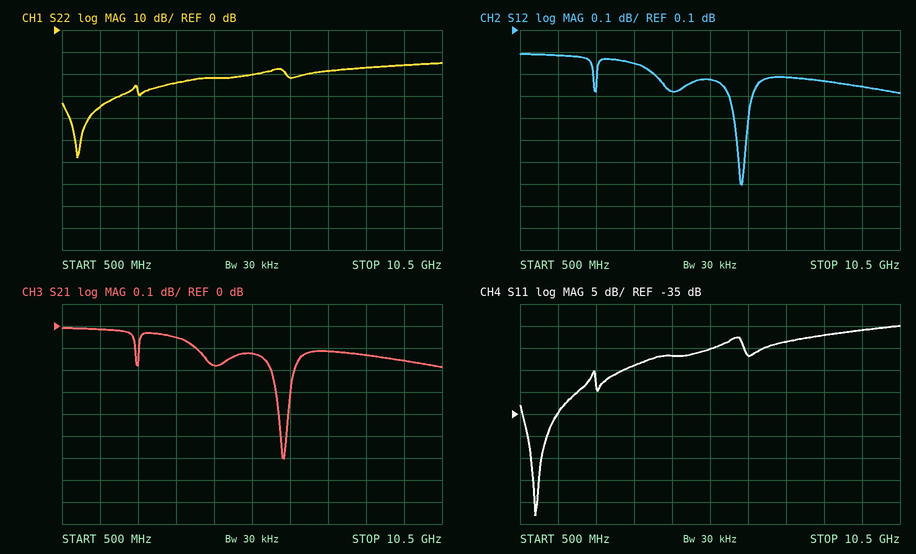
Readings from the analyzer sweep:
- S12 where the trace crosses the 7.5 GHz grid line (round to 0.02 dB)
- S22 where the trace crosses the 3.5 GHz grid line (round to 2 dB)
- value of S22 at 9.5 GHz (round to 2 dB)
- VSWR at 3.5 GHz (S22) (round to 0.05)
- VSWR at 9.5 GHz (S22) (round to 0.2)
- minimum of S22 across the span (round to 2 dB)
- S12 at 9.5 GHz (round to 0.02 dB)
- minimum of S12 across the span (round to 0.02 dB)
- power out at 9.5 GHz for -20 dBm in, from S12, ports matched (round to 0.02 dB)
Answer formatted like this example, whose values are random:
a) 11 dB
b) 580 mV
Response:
a) -0.12 dB
b) -24 dB
c) -16 dB
d) 1.15
e) 1.4
f) -58 dB
g) -0.16 dB
h) -0.60 dB
i) -20.16 dBm
